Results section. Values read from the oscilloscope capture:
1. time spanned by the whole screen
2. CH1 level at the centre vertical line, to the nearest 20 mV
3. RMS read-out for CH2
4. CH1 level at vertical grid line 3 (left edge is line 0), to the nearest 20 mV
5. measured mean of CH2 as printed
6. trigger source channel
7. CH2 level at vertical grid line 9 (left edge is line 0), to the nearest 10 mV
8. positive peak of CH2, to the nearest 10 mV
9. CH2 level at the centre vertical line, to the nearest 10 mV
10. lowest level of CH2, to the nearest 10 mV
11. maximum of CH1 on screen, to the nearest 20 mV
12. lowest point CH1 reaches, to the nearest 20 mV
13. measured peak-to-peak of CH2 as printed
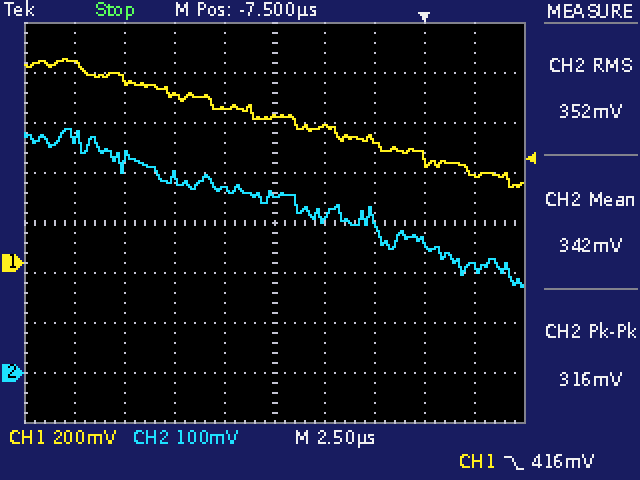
25 µs
580 mV
352 mV
680 mV
342 mV
CH1
210 mV
490 mV
360 mV
170 mV
820 mV
300 mV
316 mV
